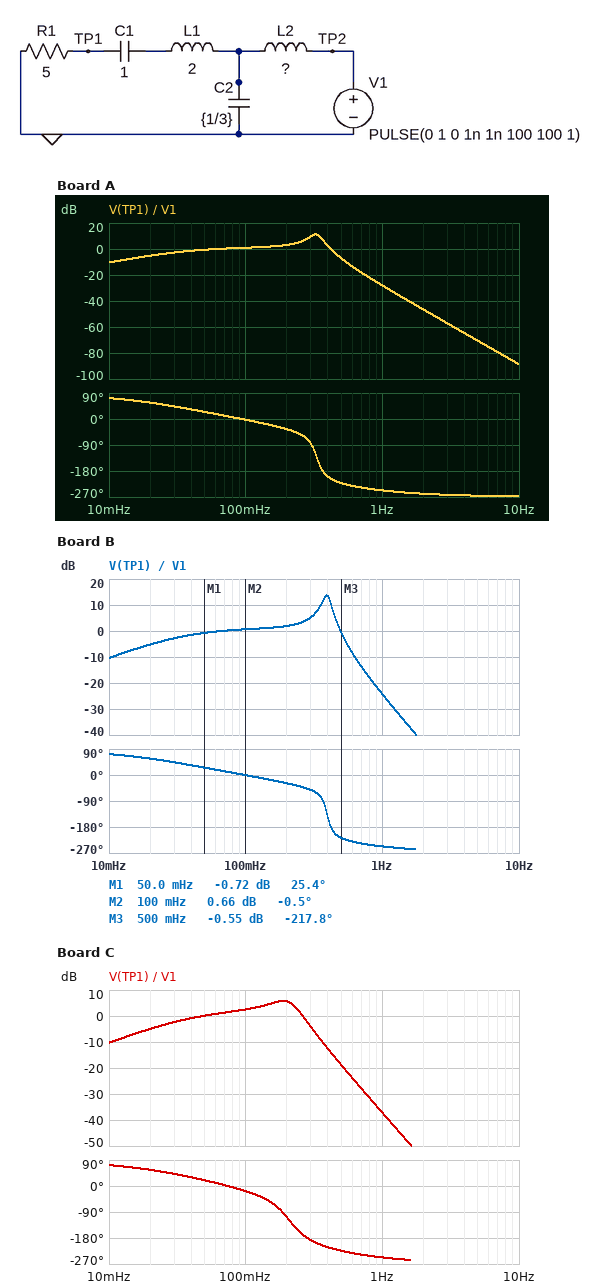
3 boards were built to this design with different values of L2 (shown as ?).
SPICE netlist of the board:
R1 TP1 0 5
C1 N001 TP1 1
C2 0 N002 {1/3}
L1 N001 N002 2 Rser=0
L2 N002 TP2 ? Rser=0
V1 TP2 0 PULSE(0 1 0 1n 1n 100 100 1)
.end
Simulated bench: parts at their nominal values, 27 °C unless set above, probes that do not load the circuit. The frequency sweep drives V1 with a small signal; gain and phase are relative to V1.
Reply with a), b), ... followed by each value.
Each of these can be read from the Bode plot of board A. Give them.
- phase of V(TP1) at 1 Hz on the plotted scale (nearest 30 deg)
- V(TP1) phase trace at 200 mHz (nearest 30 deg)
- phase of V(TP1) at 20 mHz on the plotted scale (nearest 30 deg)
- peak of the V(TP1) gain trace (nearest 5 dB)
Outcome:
a) -240 deg
b) -30 deg
c) 60 deg
d) 10 dB
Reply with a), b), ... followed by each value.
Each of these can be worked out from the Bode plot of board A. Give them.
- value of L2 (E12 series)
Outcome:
a) 820 mH
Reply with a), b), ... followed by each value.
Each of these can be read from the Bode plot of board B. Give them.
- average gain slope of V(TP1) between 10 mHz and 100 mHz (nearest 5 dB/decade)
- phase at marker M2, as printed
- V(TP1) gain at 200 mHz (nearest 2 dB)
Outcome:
a) 10 dB/decade
b) -0.5 deg
c) 2 dB
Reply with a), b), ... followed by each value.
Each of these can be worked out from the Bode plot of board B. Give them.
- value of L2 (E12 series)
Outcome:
a) 560 mH
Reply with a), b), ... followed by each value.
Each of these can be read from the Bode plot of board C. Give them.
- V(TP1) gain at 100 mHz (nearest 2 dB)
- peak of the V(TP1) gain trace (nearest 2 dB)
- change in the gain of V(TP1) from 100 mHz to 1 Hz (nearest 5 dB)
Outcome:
a) 2 dB
b) 6 dB
c) -40 dB
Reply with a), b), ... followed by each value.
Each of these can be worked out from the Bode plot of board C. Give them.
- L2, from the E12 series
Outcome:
a) 2.2 H
